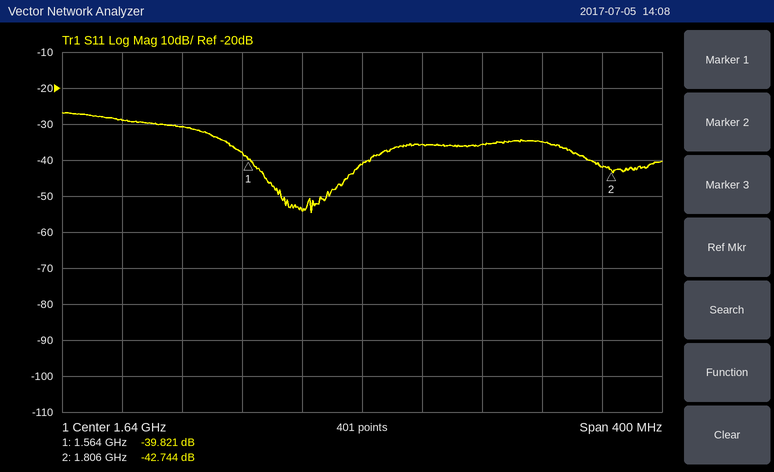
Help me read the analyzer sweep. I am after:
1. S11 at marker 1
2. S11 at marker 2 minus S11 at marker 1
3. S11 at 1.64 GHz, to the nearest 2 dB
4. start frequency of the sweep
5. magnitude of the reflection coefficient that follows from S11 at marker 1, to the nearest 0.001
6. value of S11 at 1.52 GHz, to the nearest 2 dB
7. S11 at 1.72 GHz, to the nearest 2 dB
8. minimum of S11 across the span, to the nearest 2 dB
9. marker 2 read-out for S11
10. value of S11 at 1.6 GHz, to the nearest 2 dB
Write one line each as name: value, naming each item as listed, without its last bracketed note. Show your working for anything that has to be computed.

S11 at marker 1: -39.821 dB
S11 at marker 2 minus S11 at marker 1: -42.744 − (-39.821) = -2.923 dB
S11 at 1.64 GHz, to the nearest 2 dB: -42 dB
start frequency of the sweep: 1.44 GHz
magnitude of the reflection coefficient that follows from S11 at marker 1, to the nearest 0.001: 10^(-39.821/20) ≈ 0.010
value of S11 at 1.52 GHz, to the nearest 2 dB: -30 dB
S11 at 1.72 GHz, to the nearest 2 dB: -36 dB
minimum of S11 across the span, to the nearest 2 dB: -54 dB
marker 2 read-out for S11: -42.744 dB
value of S11 at 1.6 GHz, to the nearest 2 dB: -54 dB
